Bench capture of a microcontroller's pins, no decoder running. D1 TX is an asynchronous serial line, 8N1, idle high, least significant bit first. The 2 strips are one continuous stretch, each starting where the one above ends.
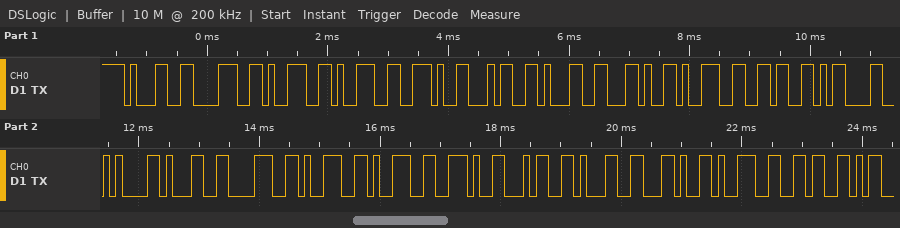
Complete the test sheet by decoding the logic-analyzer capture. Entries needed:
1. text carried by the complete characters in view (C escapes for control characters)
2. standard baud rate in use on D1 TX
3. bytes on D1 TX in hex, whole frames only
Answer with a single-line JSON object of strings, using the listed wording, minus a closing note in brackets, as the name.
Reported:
{"text carried by the complete characters in view": "\"1899.41,96\\r\\n1899.41,96\"", "standard baud rate in use on D1 TX": "9600 baud", "bytes on D1 TX in hex, whole frames only": "31 38 39 39 2E 34 31 2C 39 36 0D 0A 31 38 39 39 2E 34 31 2C 39 36"}
